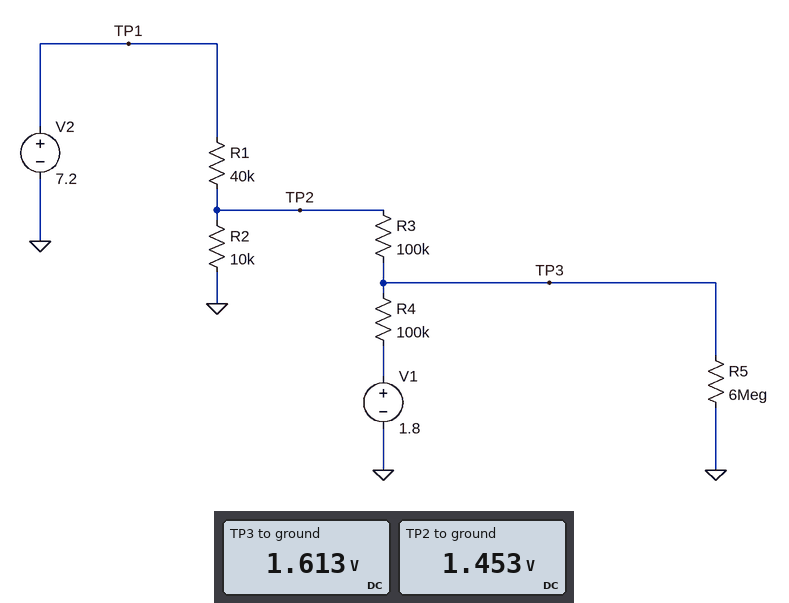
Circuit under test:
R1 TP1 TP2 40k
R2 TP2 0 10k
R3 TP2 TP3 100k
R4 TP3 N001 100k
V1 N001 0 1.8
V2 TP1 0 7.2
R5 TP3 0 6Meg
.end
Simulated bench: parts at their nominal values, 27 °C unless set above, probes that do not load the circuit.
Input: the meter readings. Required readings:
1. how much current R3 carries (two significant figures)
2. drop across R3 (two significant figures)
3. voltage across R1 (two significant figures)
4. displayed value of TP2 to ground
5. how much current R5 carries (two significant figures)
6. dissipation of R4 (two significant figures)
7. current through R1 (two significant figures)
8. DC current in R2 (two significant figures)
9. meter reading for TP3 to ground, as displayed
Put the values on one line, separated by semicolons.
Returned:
1.6 µA; 160 mV; 5.7 V; 1.453 V; 270 nA; 350 nW; 140 µA; 150 µA; 1.613 V
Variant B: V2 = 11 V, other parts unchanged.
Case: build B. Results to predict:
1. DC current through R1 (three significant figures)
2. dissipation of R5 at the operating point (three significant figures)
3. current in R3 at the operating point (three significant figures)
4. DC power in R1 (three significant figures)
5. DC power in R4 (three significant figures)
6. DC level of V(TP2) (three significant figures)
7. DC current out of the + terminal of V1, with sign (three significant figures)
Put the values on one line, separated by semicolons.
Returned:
220 µA; 650 nW; 2.08 µA; 1.94 mW; 307 nW; 2.18 V; -1.75 µA
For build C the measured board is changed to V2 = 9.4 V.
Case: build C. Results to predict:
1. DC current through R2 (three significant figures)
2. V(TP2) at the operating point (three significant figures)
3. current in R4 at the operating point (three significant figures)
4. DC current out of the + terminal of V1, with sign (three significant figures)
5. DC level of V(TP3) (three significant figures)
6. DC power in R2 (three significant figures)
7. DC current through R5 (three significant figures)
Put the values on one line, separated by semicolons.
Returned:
188 µA; 1.88 V; 227 nA; -227 nA; 1.82 V; 352 µW; 304 nA
